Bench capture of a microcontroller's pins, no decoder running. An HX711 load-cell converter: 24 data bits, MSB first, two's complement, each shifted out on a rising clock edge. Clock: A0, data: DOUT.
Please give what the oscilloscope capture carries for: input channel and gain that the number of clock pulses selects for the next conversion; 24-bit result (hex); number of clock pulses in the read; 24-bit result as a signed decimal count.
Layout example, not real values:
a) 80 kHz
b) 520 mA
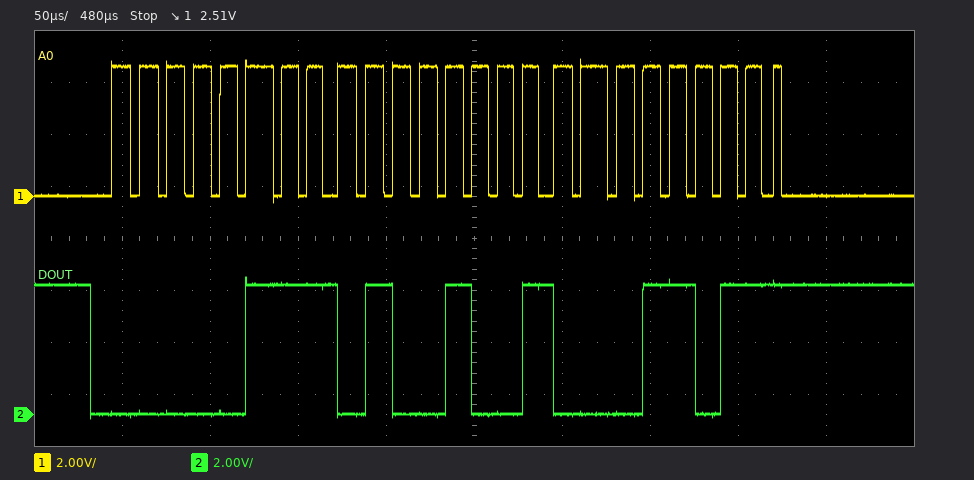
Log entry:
a) channel A, gain 128
b) 0x07491B
c) 25
d) 477467
